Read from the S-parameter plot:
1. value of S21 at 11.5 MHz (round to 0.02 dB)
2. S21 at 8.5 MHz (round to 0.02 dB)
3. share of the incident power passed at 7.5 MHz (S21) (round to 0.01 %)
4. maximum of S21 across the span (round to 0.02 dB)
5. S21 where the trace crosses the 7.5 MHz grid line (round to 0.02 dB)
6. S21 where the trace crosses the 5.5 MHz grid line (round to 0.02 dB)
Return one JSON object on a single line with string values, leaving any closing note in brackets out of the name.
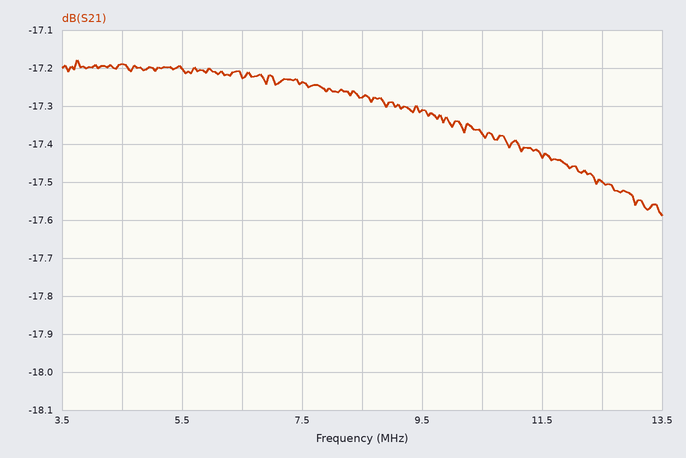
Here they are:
{"value of S21 at 11.5 MHz": "-17.44 dB", "S21 at 8.5 MHz": "-17.28 dB", "share of the incident power passed at 7.5 MHz (S21)": "1.89 %", "maximum of S21 across the span": "-17.18 dB", "S21 where the trace crosses the 7.5 MHz grid line": "-17.24 dB", "S21 where the trace crosses the 5.5 MHz grid line": "-17.20 dB"}
